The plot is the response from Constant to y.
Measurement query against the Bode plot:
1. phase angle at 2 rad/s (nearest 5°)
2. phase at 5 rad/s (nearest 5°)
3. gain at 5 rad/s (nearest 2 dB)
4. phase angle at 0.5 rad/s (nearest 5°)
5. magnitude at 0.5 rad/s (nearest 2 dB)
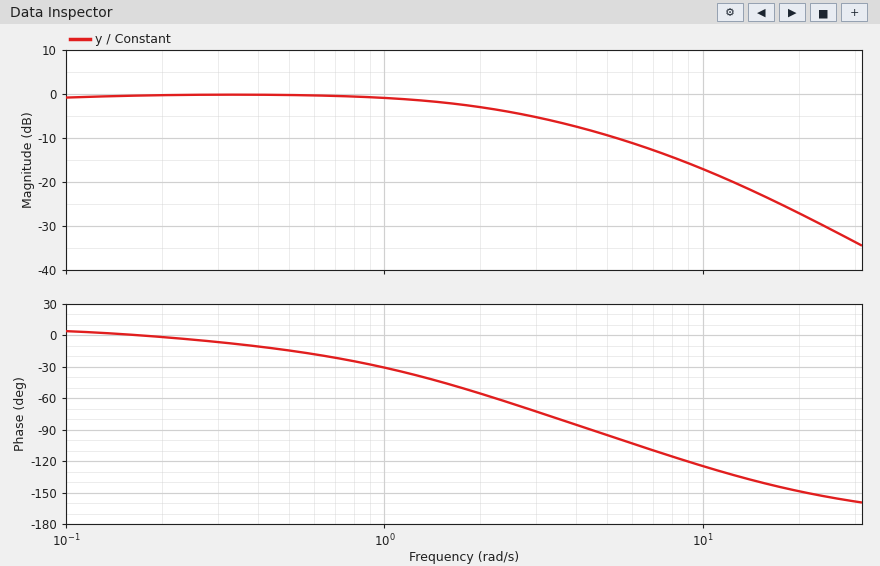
-55°
-95°
-10 dB
-15°
0 dB
